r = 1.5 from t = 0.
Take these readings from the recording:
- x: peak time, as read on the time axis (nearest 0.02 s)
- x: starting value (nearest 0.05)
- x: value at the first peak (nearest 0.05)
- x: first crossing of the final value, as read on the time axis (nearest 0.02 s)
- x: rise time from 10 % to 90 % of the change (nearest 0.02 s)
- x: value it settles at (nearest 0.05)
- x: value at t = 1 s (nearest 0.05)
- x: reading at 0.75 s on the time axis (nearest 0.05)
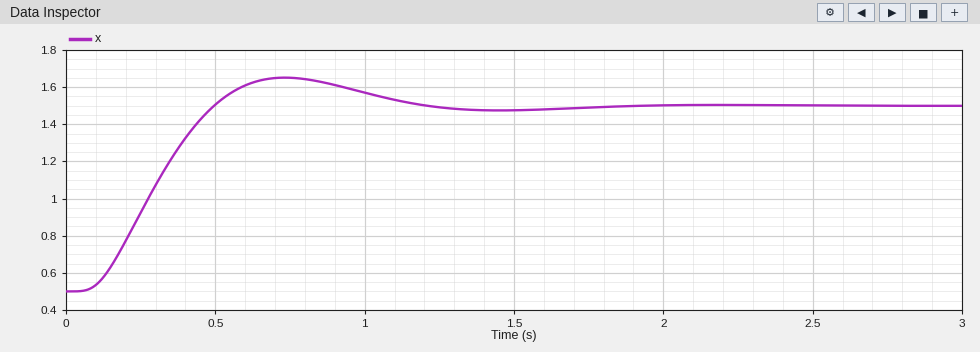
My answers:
0.74 s
0.50
1.65
0.50 s
0.30 s
1.50
1.55
1.65
